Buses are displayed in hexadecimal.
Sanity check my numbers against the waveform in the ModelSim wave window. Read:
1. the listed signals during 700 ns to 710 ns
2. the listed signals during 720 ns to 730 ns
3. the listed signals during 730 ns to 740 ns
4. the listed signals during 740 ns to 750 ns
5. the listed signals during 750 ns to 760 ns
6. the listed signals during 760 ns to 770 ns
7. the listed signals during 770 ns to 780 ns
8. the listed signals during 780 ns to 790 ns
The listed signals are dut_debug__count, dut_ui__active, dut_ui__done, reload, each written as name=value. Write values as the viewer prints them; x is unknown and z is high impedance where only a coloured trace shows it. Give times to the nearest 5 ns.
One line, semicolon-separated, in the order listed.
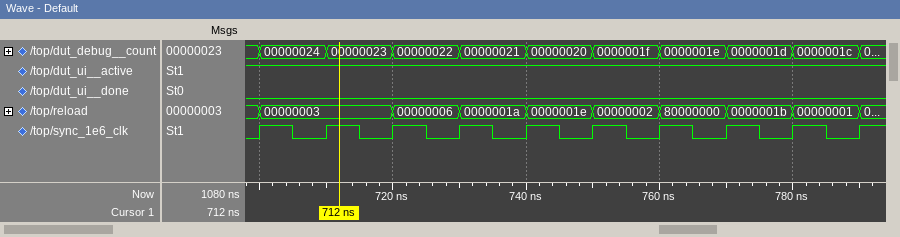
dut_debug__count=00000024, dut_ui__active=1, dut_ui__done=0, reload=00000003; dut_debug__count=00000022, dut_ui__active=1, dut_ui__done=0, reload=00000006; dut_debug__count=00000021, dut_ui__active=1, dut_ui__done=0, reload=0000001a; dut_debug__count=00000020, dut_ui__active=1, dut_ui__done=0, reload=0000001e; dut_debug__count=0000001f, dut_ui__active=1, dut_ui__done=0, reload=00000002; dut_debug__count=0000001e, dut_ui__active=1, dut_ui__done=0, reload=80000000; dut_debug__count=0000001d, dut_ui__active=1, dut_ui__done=0, reload=0000001b; dut_debug__count=0000001c, dut_ui__active=1, dut_ui__done=0, reload=00000001
